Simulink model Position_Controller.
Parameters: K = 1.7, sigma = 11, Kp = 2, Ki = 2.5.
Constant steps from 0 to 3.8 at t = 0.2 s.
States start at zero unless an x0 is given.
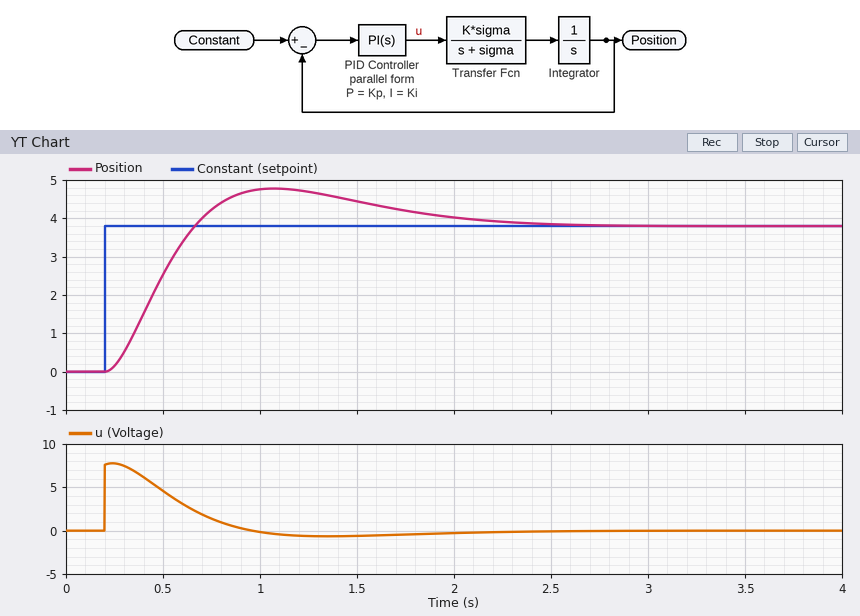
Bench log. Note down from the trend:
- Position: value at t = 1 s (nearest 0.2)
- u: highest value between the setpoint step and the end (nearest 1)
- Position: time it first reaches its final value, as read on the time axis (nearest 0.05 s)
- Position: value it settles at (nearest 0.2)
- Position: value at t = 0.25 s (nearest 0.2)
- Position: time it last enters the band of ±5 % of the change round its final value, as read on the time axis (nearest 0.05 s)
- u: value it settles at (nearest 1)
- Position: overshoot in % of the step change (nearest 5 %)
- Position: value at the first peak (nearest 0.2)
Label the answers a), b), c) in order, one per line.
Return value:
a) 4.8
b) 8
c) 0.65 s
d) 3.8
e) 0.2
f) 2.05 s
g) 0
h) 25 %
i) 4.8
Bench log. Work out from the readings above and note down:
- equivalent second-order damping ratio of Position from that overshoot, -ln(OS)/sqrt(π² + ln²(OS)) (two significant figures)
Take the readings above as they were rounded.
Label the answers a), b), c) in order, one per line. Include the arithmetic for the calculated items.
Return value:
a) ln(0.25) = -1.386; 1.386 / sqrt(9.870 + 1.922) = 0.40
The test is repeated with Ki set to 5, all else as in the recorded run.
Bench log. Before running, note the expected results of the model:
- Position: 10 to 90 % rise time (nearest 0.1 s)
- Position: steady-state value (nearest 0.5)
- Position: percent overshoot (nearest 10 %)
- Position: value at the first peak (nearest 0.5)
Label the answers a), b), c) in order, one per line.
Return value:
a) 0.3 s
b) 4.0
c) 40 %
d) 5.5
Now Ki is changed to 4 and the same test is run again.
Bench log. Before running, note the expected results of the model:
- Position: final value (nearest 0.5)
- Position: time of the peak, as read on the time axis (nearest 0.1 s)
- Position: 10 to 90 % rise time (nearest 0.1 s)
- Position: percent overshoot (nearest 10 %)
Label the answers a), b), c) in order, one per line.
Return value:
a) 4.0
b) 1.0 s
c) 0.3 s
d) 40 %
